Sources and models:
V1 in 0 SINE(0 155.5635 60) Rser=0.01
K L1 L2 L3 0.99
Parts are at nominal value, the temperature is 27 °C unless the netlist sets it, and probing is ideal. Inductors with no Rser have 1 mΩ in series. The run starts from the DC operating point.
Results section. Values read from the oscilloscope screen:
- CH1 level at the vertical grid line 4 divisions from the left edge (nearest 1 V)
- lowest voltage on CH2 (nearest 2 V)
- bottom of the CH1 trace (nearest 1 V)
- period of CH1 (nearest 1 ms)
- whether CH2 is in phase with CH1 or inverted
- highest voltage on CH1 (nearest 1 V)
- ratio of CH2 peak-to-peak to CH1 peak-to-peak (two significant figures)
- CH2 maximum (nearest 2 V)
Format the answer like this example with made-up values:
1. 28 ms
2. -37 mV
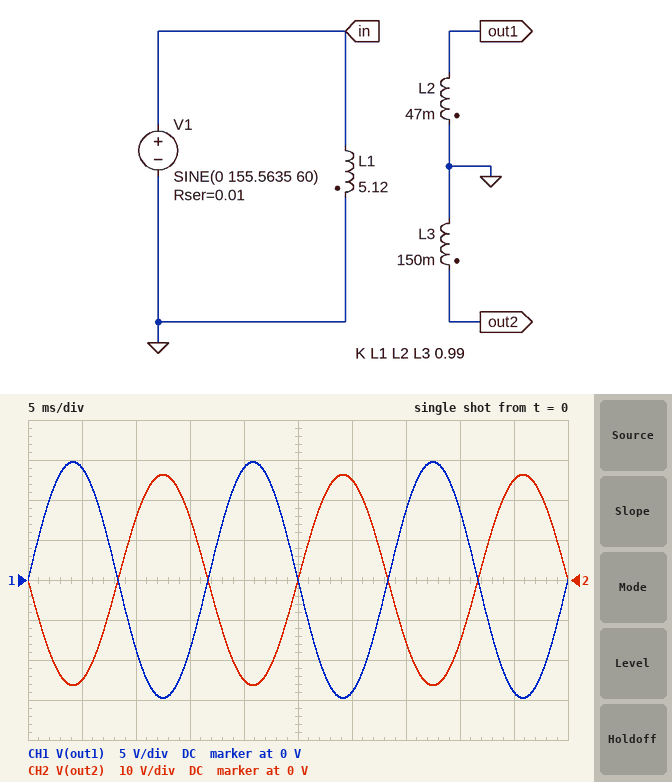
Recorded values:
1. 14 V
2. -26 V
3. -15 V
4. 17 ms
5. inverted
6. 15 V
7. 1.8
8. 26 V
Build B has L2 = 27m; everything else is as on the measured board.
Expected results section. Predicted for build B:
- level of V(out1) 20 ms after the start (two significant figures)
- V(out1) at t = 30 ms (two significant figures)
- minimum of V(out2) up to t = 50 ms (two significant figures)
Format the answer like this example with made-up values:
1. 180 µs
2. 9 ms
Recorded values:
1. 11 V
2. -11 V
3. -26 V
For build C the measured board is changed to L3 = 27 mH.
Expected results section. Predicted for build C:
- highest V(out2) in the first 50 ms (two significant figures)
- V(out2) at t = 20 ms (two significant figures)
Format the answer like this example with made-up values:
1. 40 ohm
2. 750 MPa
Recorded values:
1. 11 V
2. -11 V
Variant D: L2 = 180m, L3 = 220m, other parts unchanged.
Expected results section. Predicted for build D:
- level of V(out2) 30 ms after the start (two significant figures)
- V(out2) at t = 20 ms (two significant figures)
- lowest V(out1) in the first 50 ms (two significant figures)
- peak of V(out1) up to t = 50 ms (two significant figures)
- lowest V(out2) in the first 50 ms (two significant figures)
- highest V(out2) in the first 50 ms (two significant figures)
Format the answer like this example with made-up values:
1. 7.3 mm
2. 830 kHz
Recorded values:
1. 30 V
2. -30 V
3. -29 V
4. 29 V
5. -32 V
6. 32 V
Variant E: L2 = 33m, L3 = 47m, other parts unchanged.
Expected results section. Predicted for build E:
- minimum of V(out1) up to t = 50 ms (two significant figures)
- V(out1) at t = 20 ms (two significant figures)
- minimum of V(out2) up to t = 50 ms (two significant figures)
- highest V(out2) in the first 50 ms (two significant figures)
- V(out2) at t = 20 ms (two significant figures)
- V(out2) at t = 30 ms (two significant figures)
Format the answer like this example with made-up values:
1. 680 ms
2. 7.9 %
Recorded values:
1. -12 V
2. 12 V
3. -15 V
4. 15 V
5. -14 V
6. 14 V
